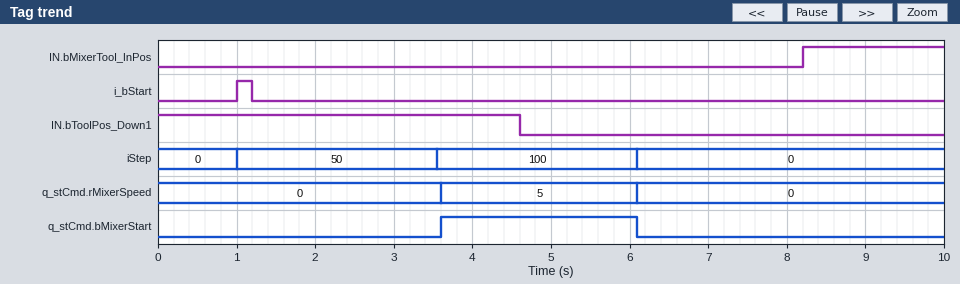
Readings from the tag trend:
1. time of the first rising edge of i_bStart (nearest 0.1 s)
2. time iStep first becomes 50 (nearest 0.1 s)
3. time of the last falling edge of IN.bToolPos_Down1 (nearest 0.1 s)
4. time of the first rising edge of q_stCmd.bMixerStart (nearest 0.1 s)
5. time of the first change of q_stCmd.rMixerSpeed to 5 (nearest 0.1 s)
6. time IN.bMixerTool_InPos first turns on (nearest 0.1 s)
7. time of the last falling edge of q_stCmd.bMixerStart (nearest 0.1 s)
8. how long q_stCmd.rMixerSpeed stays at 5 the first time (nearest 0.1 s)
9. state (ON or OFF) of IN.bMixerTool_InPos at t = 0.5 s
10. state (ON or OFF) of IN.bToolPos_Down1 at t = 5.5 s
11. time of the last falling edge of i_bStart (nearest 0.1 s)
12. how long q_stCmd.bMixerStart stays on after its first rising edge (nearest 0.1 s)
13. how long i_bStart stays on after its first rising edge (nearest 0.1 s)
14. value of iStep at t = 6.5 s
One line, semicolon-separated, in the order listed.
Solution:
1.0 s; 1.0 s; 4.6 s; 3.6 s; 3.6 s; 8.2 s; 6.1 s; 2.5 s; OFF; OFF; 1.2 s; 2.5 s; 0.2 s; 0
